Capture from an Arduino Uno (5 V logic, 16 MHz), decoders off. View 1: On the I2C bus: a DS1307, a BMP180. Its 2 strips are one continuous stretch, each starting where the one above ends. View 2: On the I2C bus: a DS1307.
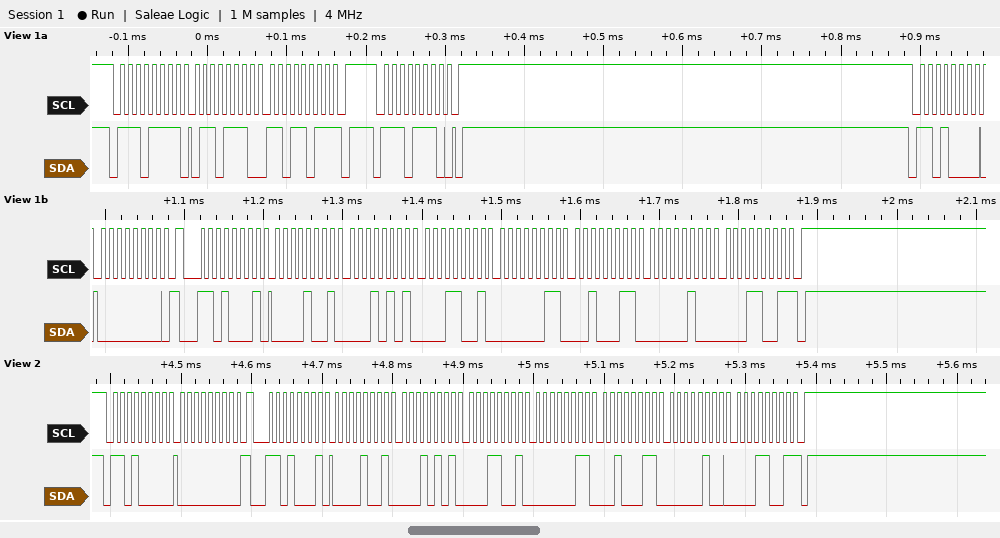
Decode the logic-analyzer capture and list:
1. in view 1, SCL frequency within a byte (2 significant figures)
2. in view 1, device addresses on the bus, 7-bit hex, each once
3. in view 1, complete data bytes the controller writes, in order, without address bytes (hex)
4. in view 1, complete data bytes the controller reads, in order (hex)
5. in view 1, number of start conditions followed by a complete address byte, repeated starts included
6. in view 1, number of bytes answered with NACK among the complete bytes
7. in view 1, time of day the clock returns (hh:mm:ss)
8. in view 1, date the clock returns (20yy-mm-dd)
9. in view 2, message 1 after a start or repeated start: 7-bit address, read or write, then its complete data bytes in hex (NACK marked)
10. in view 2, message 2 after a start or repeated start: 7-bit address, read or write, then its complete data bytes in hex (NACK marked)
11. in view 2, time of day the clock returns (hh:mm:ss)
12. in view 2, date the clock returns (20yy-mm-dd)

100 kHz
0x77 0x68
00
6E DB 09 15 19 03 23 04 19
4
2
19:15:09
2019-04-23
0x68 write: 00
0x68 read: 09 15 19 03 23 04 19 NACK
19:15:09
2019-04-23
